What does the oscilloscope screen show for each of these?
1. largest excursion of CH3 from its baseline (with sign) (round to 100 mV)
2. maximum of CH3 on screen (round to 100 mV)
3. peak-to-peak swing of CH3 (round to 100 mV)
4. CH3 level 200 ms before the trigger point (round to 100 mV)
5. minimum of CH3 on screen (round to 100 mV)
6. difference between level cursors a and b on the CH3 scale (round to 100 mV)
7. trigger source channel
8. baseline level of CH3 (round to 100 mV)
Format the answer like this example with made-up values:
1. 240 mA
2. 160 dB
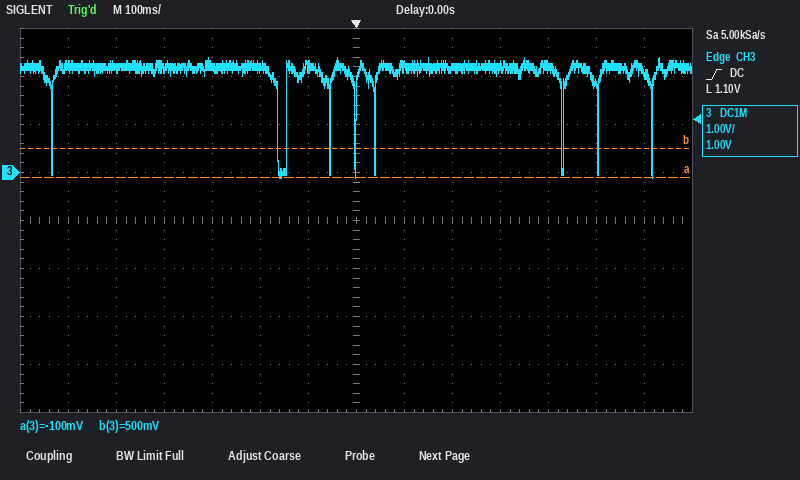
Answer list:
1. -2.3 V
2. 2.4 V
3. 2.5 V
4. 2.2 V
5. -100 mV
6. 600 mV
7. CH3
8. 2.2 V
